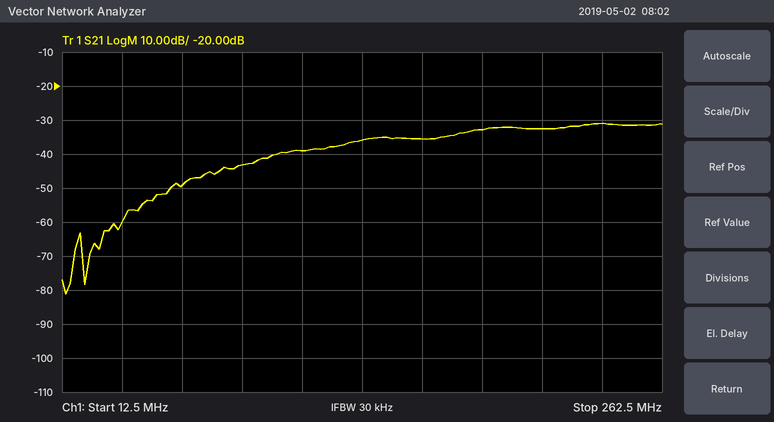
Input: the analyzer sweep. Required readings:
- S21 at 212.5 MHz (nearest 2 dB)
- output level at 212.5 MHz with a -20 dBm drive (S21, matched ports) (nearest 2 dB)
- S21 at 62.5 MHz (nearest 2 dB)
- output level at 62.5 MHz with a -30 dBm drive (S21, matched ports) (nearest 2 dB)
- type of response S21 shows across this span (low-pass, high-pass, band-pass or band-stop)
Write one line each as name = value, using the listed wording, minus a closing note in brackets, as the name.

S21 at 212.5 MHz = -32 dB
output level at 212.5 MHz with a -20 dBm drive (S21, matched ports) = -52 dBm
S21 at 62.5 MHz = -50 dB
output level at 62.5 MHz with a -30 dBm drive (S21, matched ports) = -80 dBm
type of response S21 shows across this span = high-pass
